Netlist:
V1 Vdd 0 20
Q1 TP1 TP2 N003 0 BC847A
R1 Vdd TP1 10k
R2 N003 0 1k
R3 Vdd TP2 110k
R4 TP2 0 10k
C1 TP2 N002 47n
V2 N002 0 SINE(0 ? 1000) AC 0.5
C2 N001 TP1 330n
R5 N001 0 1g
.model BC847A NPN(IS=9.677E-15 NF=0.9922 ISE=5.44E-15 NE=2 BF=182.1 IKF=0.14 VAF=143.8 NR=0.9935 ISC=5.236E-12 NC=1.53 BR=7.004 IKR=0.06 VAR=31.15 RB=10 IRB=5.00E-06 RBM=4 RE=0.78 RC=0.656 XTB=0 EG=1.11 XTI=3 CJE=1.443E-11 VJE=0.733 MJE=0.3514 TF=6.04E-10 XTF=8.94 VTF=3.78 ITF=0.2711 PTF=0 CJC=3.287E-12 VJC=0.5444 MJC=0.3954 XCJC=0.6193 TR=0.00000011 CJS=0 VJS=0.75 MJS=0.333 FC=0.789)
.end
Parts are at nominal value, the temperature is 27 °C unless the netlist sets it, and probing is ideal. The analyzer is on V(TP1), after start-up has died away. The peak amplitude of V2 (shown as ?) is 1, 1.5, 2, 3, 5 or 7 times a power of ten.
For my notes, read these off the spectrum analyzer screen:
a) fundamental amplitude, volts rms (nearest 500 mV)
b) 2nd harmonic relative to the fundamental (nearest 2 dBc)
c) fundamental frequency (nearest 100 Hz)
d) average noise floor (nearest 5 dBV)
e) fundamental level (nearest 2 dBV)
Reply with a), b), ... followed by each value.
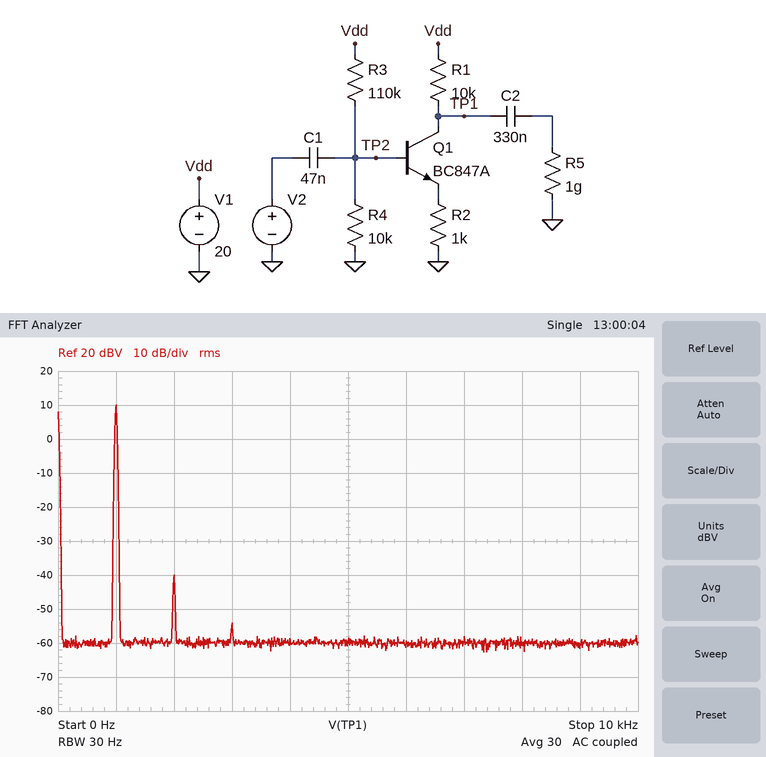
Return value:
a) 3.0 V
b) -50 dBc
c) 1.0 kHz
d) -60 dBV
e) 10 dBV
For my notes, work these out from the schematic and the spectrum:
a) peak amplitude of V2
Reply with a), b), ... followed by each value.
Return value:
a) 500 mV
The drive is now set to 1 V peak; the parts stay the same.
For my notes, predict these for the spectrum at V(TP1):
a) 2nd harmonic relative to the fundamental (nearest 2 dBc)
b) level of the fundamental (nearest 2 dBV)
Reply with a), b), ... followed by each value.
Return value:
a) -42 dBc
b) 16 dBV
